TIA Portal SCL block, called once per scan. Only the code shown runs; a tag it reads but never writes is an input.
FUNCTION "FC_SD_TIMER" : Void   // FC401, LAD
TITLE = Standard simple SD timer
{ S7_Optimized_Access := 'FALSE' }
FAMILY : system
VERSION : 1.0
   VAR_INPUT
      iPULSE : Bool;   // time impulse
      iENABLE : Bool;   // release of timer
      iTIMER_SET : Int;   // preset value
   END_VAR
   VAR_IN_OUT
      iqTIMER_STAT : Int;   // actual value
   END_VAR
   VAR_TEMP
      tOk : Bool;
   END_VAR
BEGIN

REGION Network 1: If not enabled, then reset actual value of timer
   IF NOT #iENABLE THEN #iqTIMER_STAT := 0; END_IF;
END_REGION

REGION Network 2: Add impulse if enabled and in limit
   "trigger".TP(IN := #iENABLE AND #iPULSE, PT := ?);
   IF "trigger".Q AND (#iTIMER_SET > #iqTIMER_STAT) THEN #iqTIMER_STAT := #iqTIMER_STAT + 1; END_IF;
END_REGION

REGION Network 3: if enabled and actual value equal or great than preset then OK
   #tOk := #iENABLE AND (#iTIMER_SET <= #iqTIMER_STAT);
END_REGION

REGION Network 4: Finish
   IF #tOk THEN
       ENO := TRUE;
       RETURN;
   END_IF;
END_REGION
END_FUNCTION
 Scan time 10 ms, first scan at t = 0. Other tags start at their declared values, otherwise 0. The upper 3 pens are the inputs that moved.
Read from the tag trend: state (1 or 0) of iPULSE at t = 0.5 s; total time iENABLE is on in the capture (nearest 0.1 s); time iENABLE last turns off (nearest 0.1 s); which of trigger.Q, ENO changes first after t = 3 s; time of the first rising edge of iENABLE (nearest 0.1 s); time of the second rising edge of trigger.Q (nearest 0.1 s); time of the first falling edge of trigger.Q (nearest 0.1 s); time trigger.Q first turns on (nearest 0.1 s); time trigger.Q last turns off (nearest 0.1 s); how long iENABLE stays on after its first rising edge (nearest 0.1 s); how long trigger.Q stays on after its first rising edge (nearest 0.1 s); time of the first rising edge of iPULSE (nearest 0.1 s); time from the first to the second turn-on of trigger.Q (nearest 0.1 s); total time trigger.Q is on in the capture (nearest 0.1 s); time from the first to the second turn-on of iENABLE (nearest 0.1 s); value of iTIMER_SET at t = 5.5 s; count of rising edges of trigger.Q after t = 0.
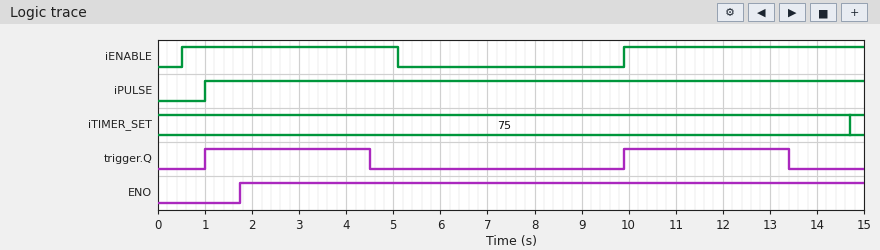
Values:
0
9.7 s
5.1 s
trigger.Q
0.5 s
9.9 s
4.5 s
1.0 s
13.4 s
4.6 s
3.5 s
1.0 s
8.9 s
7.0 s
9.4 s
75
2
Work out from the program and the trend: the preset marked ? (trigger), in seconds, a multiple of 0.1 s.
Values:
3.5 s
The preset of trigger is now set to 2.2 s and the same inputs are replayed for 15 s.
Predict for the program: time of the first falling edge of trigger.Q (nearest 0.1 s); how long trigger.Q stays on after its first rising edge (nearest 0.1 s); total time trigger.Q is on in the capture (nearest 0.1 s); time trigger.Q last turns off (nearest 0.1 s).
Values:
3.2 s
2.2 s
4.4 s
12.1 s
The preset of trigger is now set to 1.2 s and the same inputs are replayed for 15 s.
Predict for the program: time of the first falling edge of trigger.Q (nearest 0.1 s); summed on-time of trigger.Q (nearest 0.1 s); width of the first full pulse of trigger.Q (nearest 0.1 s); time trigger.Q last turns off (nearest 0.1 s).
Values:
2.2 s
2.4 s
1.2 s
11.1 s
